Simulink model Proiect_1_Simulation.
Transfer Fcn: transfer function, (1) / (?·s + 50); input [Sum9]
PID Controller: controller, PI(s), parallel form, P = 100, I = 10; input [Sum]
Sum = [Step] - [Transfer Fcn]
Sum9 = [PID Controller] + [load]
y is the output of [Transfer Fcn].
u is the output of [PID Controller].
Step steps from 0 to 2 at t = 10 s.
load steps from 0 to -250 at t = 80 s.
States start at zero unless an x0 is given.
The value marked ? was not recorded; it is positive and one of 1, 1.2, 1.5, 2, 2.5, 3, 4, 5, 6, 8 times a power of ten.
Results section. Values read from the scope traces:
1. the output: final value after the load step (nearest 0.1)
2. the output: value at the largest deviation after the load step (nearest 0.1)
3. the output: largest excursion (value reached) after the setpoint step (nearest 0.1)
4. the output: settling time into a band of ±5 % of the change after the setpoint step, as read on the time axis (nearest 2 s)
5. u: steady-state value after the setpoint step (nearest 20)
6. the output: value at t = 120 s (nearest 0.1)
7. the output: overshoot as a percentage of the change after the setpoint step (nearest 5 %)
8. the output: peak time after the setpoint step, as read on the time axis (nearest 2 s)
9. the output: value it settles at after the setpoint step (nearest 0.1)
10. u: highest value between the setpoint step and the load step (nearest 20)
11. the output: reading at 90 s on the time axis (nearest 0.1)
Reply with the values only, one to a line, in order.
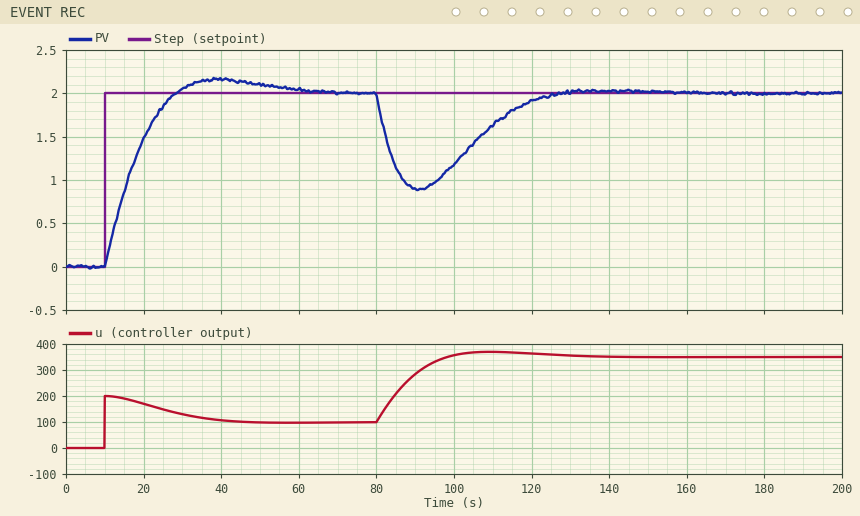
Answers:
2.0
0.9
2.2
50 s
100
1.9
10 %
40 s
2.0
200
0.9
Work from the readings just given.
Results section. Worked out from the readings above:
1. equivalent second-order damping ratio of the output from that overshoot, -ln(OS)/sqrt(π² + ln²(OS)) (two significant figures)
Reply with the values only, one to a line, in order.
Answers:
0.59
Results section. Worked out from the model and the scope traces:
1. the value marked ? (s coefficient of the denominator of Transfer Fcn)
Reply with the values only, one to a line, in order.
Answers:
1000
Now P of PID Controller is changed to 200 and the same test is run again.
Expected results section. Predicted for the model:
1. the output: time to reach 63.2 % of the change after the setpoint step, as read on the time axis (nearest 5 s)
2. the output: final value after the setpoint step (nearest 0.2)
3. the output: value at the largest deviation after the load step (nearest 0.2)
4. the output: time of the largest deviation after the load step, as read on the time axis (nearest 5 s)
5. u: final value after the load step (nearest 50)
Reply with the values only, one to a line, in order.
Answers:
15 s
2.0
1.2
90 s
350
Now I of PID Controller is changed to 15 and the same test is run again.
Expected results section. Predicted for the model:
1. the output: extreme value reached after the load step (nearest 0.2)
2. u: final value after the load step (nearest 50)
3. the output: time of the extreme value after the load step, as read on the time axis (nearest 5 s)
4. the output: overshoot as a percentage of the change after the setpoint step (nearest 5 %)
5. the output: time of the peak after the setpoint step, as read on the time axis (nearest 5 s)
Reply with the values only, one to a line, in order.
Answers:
1.0
350
90 s
15 %
35 s
